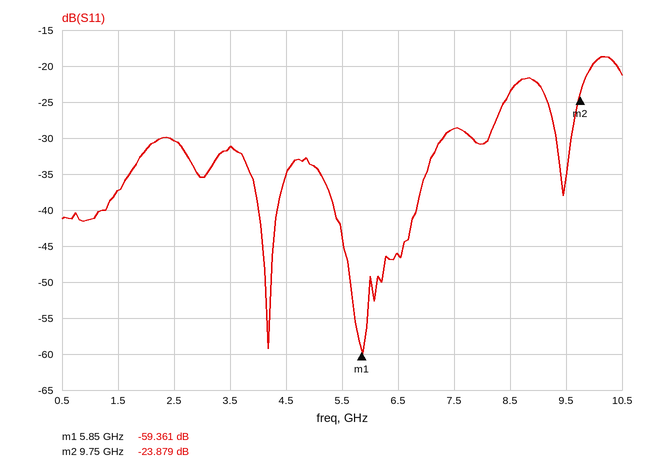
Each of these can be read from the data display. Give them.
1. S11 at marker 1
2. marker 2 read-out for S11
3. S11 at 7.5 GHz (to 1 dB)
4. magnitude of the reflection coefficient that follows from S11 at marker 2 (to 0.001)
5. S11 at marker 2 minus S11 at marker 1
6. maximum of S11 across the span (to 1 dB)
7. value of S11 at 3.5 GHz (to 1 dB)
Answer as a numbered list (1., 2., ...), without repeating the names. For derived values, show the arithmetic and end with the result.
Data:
1. -59.361 dB
2. -23.879 dB
3. -29 dB
4. 10^(-23.879/20) ≈ 0.064
5. -23.879 − (-59.361) = 35.482 dB
6. -19 dB
7. -31 dB
